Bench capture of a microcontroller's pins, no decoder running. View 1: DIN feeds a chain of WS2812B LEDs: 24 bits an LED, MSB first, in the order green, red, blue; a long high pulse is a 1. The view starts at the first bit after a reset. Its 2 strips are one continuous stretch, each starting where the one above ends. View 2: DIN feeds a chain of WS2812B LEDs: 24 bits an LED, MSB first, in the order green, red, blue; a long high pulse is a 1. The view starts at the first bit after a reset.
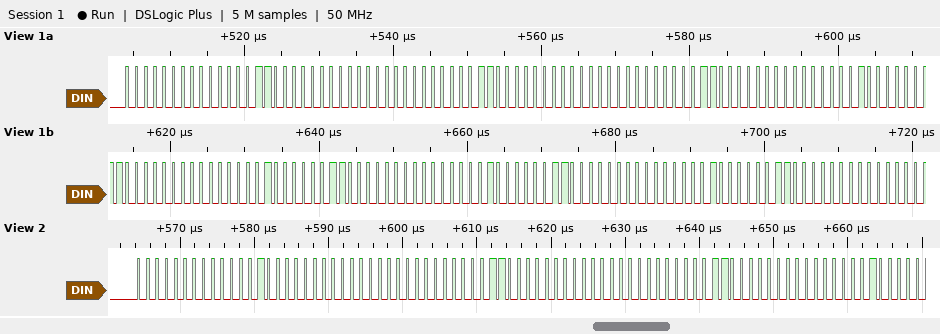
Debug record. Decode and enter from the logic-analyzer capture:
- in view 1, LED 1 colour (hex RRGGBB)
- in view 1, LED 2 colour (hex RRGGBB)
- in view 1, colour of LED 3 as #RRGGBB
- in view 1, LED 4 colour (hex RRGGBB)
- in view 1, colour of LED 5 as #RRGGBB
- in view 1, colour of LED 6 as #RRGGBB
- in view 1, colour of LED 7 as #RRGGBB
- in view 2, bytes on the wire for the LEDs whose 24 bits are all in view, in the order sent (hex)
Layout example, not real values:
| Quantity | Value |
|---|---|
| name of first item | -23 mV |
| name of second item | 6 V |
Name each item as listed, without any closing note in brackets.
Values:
| Quantity | Value |
|---|---|
| in view 1, LED 1 colour | #030000 |
| in view 1, LED 2 colour | #030000 |
| in view 1, colour of LED 3 as #RRGGBB | #030000 |
| in view 1, LED 4 colour | #030100 |
| in view 1, colour of LED 5 as #RRGGBB | #030100 |
| in view 1, colour of LED 6 as #RRGGBB | #030100 |
| in view 1, colour of LED 7 as #RRGGBB | #030100 |
| in view 2, bytes on the wire for the LEDs whose 24 bits are all in view, in the order sent | 00 04 00 00 03 00 00 03 00 |
